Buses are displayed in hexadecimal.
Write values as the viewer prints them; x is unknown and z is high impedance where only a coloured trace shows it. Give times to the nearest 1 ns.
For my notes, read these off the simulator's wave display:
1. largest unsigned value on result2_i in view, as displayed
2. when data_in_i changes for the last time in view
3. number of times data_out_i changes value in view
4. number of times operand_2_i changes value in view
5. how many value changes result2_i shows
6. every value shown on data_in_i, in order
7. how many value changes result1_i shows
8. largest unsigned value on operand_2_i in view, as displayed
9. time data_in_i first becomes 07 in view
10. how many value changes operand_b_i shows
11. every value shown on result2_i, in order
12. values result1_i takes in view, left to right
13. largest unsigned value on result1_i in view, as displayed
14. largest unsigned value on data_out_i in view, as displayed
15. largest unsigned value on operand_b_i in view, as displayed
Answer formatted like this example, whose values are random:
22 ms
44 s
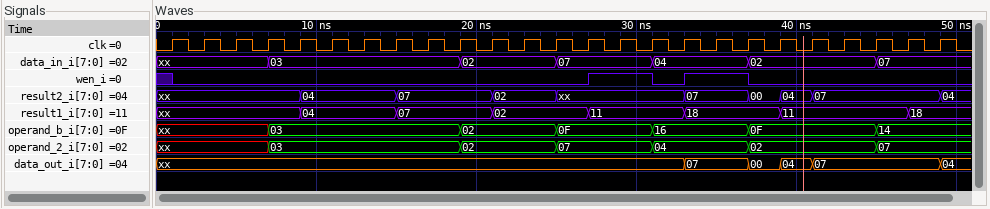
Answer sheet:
07
45 ns
5
6
9
xx, 03, 02, 07, 04, 02, 07
7
07
25 ns
6
xx, 04, 07, 02, xx, 07, 00, 04, 07, 04
xx, 04, 07, 02, 11, 18, 11, 18
18
07
16
